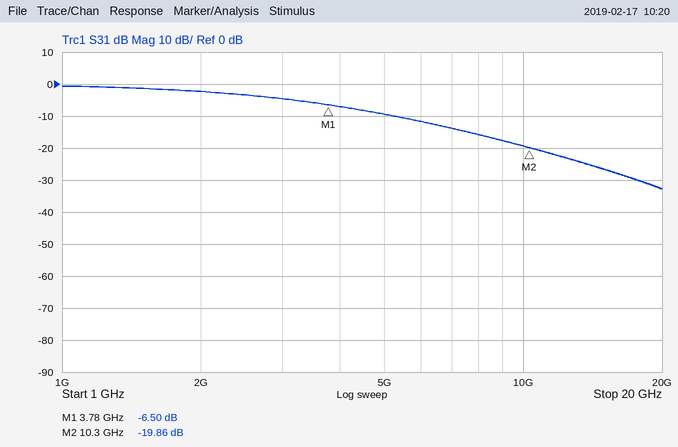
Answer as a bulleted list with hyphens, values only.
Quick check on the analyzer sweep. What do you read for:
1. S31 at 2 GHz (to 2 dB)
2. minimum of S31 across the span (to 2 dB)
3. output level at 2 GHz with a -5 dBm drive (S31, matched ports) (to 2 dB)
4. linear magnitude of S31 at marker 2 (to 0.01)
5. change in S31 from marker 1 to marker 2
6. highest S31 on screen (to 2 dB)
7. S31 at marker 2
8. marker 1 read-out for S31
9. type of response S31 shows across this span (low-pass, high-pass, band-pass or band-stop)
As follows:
- -2 dB
- -32 dB
- -8 dBm
- 0.10
- -13.36 dB
- 0 dB
- -19.86 dB
- -6.50 dB
- low-pass
